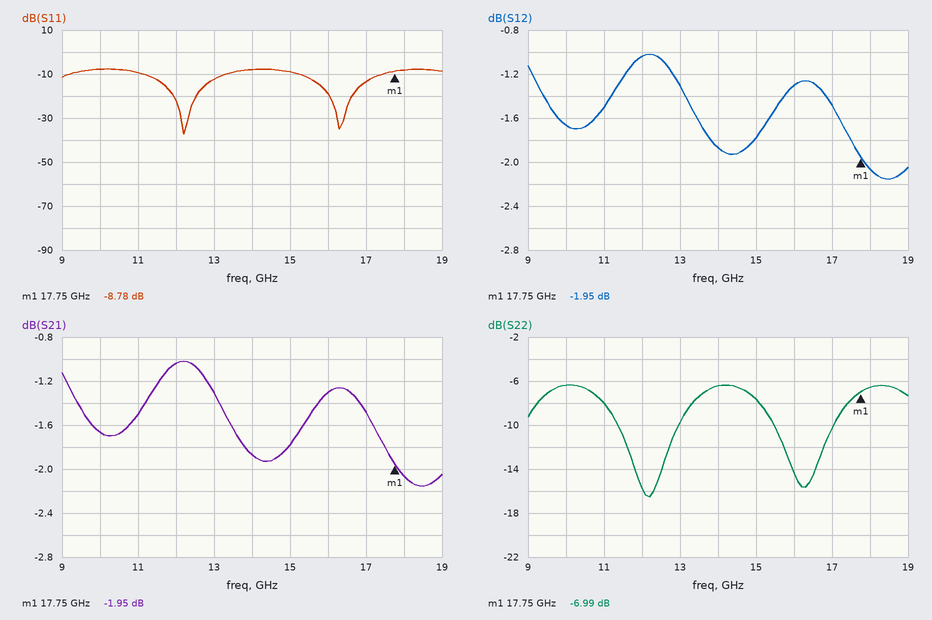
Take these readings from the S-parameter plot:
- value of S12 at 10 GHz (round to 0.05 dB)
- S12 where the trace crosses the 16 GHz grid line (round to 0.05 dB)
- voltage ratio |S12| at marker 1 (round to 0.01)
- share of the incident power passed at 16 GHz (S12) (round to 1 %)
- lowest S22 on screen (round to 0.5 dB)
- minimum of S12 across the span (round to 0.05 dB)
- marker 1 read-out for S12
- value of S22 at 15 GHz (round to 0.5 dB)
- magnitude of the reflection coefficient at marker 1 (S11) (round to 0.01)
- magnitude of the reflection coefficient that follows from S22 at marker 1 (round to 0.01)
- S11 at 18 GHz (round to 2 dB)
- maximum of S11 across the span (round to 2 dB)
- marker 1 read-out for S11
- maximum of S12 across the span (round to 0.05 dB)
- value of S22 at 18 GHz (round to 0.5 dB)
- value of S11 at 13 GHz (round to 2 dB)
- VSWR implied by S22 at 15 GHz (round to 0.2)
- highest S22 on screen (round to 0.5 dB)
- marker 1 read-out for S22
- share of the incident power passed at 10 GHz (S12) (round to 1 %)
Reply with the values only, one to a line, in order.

-1.65 dB
-1.30 dB
0.80
74 %
-16.5 dB
-2.15 dB
-1.95 dB
-7.5 dB
0.36
0.45
-8 dB
-8 dB
-8.78 dB
-1.00 dB
-6.5 dB
-12 dB
2.4
-6.5 dB
-6.99 dB
68 %
